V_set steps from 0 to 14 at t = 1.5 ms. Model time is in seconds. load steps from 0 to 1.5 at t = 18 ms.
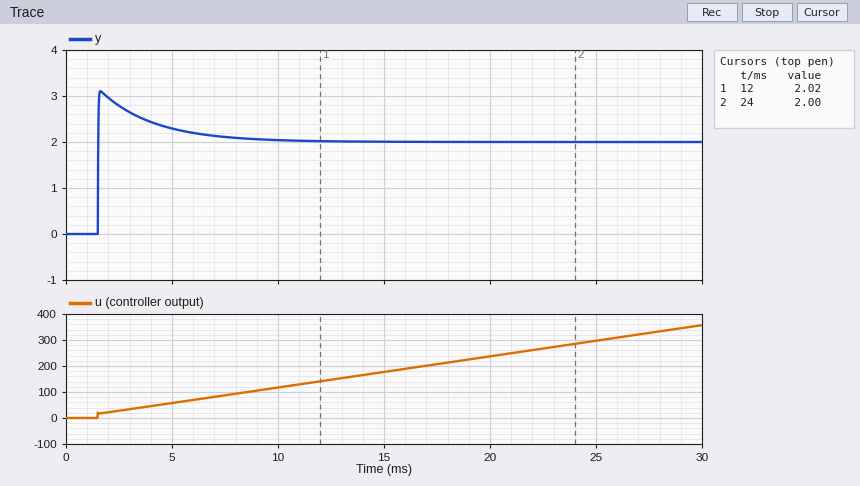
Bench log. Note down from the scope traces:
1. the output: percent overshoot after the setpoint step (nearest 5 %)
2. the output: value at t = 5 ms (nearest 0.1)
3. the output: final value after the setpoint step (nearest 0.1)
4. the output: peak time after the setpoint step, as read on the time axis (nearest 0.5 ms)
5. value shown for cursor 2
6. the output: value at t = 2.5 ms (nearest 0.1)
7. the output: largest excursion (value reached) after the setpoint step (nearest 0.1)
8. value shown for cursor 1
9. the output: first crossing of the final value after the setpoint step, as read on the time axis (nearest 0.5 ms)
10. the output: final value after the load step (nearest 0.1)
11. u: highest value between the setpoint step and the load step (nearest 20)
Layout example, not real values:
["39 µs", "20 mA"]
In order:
["55 %", "2.3", "2.0", "1.5 ms", "2.00", "2.8", "3.1", "2.02", "1.5 ms", "2.0", "220"]
